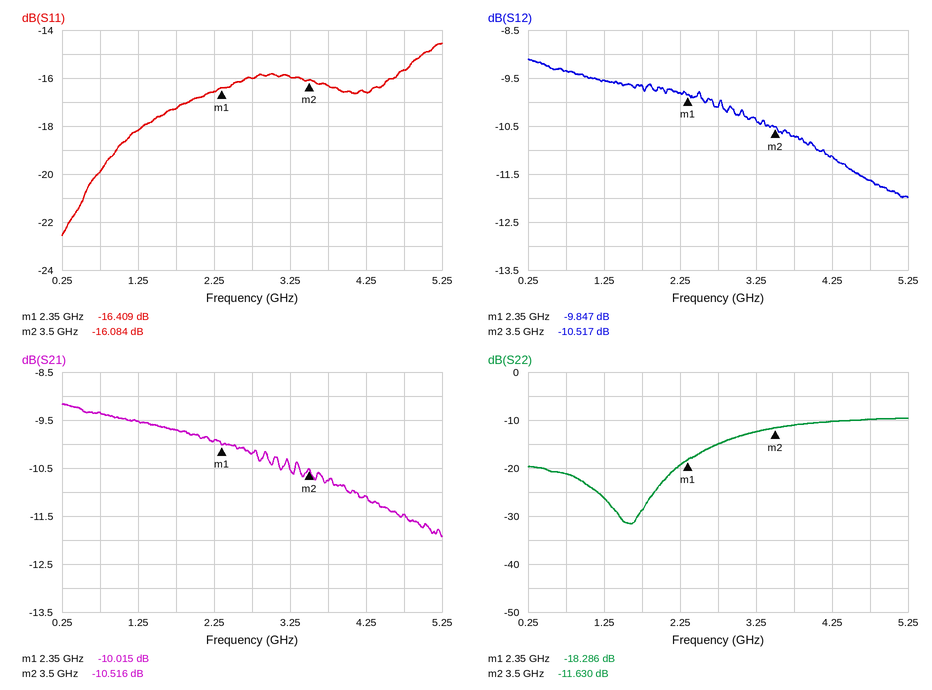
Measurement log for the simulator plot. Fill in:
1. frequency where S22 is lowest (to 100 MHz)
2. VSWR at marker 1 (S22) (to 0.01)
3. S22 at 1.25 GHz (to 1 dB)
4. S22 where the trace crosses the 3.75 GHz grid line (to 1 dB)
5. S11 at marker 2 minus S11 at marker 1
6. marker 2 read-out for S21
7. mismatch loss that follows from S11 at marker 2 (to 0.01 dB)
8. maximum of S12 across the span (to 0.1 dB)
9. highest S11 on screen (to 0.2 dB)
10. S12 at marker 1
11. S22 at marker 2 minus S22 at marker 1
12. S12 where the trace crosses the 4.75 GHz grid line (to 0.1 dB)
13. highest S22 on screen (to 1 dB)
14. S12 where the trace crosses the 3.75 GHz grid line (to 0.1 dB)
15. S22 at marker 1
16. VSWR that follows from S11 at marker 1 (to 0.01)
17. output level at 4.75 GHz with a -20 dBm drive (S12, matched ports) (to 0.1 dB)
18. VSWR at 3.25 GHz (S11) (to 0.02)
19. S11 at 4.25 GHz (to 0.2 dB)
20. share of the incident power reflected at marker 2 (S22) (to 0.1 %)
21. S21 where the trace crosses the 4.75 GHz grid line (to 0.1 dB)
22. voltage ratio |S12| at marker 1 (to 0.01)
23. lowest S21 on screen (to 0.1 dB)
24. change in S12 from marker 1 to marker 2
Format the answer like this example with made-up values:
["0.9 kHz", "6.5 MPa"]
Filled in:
["1.6 GHz", "1.28", "-26 dB", "-11 dB", "0.325 dB", "-10.516 dB", "0.11 dB", "-9.1 dB", "-14.6 dB", "-9.847 dB", "6.656 dB", "-11.6 dB", "-10 dB", "-10.7 dB", "-18.286 dB", "1.36", "-31.6 dBm", "1.38", "-16.6 dB", "6.9 %", "-11.5 dB", "0.32", "-11.9 dB", "-0.670 dB"]
